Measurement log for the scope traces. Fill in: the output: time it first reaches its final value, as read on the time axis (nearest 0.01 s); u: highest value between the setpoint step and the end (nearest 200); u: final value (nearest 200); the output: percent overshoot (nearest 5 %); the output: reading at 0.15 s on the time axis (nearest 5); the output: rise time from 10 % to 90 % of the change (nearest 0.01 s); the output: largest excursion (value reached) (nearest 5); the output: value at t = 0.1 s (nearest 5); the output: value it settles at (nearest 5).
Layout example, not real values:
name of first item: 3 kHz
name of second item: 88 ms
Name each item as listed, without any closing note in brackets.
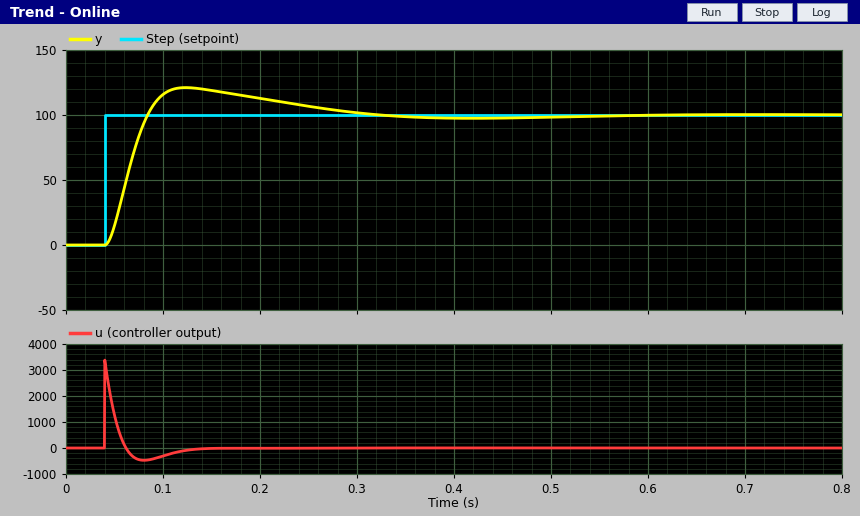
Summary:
the output: time it first reaches its final value, as read on the time axis: 0.08 s
u: highest value between the setpoint step and the end: 3400
u: final value: 0
the output: percent overshoot: 20 %
the output: reading at 0.15 s on the time axis: 120
the output: rise time from 10 % to 90 % of the change: 0.03 s
the output: largest excursion (value reached): 120
the output: value at t = 0.1 s: 115
the output: value it settles at: 100
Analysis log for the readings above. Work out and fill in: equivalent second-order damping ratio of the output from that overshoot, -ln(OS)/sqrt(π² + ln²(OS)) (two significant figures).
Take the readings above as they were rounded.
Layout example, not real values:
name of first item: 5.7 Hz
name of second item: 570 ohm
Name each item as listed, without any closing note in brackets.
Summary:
equivalent second-order damping ratio of the output from that overshoot, -ln(OS)/sqrt(π² + ln²(OS)): 0.46
